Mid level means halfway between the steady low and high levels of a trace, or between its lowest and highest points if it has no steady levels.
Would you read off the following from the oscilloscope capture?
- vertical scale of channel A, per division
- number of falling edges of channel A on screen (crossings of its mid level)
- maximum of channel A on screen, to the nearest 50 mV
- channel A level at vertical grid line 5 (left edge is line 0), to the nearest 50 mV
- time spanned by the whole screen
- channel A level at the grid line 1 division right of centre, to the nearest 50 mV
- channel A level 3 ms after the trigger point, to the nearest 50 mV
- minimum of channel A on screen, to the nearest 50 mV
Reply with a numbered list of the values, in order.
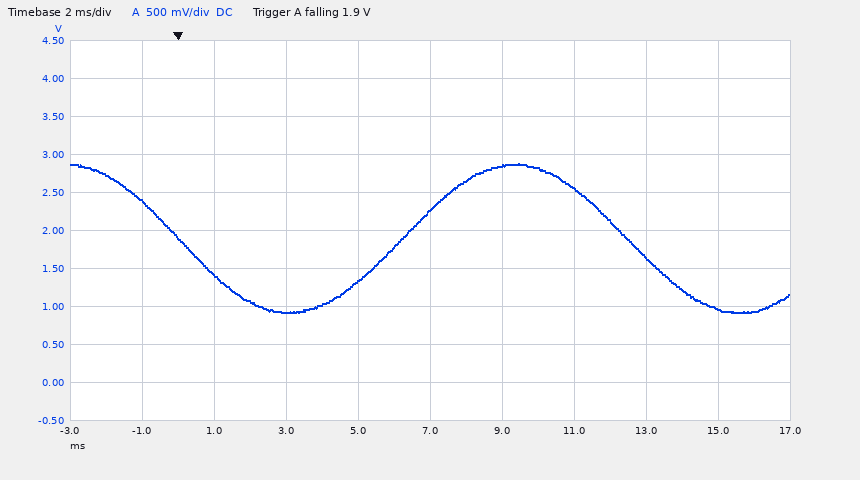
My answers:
1. 500 mV
2. 2
3. 2.90 V
4. 2.25 V
5. 20 ms
6. 2.85 V
7. 900 mV
8. 900 mV
